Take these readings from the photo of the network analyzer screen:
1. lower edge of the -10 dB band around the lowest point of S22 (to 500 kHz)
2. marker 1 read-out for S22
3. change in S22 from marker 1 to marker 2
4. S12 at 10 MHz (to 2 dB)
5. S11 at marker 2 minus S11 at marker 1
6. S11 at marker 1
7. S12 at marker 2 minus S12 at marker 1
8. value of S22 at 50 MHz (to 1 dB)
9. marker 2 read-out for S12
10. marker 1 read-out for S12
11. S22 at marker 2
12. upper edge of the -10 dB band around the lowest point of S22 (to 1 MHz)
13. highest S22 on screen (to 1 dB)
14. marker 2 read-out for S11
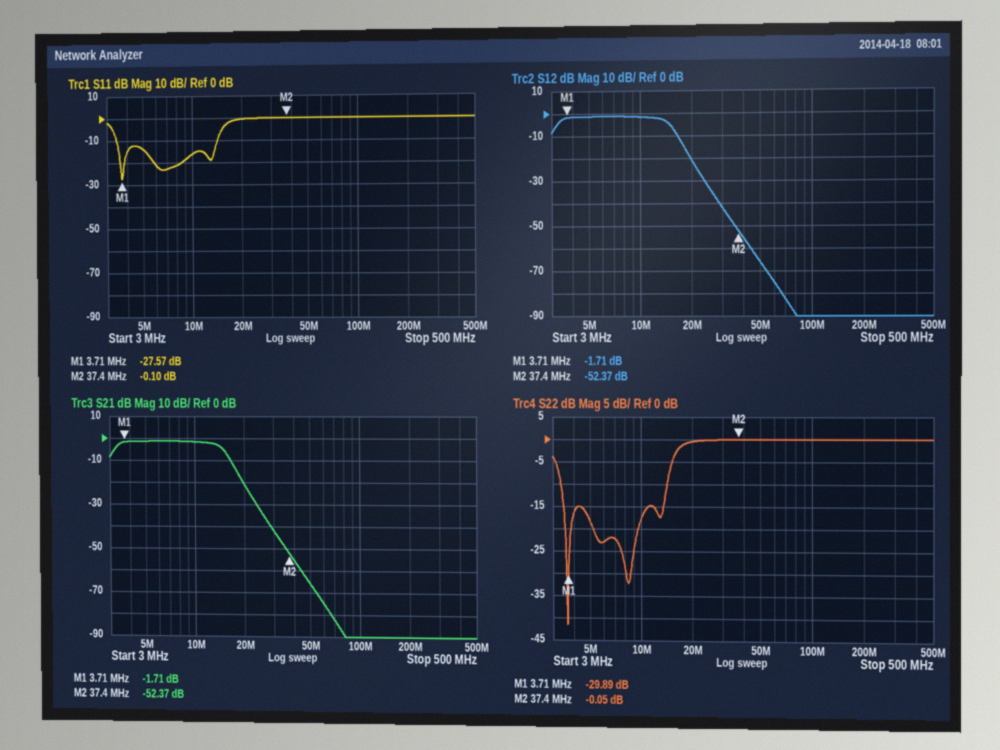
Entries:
3.5 MHz
-29.89 dB
29.84 dB
-2 dB
27.47 dB
-27.57 dB
-50.66 dB
0 dB
-52.37 dB
-1.71 dB
-0.05 dB
14 MHz
0 dB
-0.10 dB
